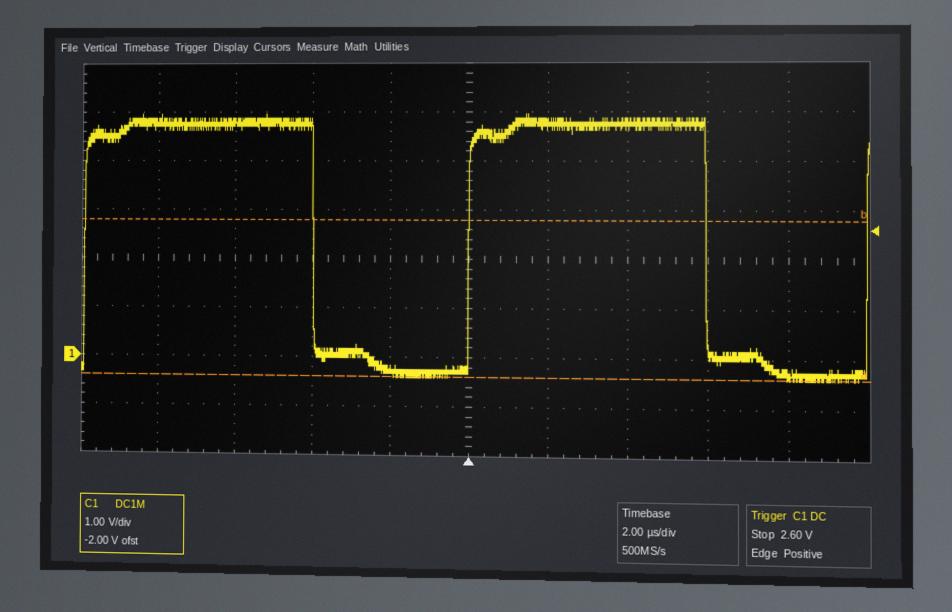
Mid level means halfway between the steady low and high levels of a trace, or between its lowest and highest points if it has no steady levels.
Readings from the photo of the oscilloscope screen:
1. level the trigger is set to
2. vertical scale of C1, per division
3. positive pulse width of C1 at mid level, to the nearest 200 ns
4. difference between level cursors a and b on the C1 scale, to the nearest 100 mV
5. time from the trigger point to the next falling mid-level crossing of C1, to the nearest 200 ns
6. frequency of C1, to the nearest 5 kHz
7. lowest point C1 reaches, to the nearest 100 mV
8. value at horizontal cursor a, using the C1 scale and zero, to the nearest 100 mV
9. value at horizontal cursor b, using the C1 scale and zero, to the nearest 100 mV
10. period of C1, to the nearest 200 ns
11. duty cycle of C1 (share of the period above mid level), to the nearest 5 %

2.60 V
1 V
6.0 µs
3.2 V
6.0 µs
100 kHz
-400 mV
-400 mV
2.8 V
10.0 µs
60 %
